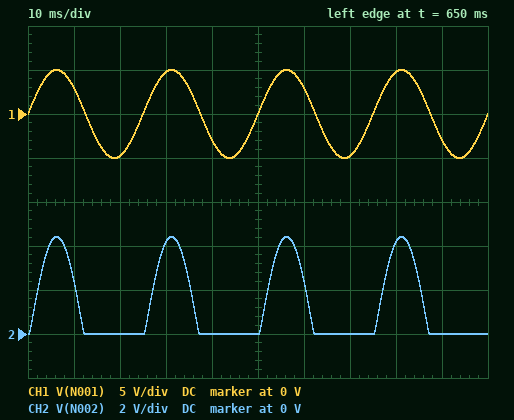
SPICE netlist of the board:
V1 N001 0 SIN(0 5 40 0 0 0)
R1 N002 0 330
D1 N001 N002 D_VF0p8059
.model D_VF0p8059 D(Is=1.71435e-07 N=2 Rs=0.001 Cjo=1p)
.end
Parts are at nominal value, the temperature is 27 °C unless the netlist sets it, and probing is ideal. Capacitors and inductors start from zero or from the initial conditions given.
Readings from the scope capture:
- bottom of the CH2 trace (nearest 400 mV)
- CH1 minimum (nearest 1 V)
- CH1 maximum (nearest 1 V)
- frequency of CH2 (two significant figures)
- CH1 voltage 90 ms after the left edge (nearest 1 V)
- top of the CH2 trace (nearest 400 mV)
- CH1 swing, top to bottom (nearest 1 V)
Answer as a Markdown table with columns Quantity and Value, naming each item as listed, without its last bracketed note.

| Quantity | Value |
|---|---|
| bottom of the CH2 trace | 0 V |
| CH1 minimum | -5 V |
| CH1 maximum | 5 V |
| frequency of CH2 | 40 Hz |
| CH1 voltage 90 ms after the left edge | -3 V |
| top of the CH2 trace | 4.4 V |
| CH1 swing, top to bottom | 10 V |
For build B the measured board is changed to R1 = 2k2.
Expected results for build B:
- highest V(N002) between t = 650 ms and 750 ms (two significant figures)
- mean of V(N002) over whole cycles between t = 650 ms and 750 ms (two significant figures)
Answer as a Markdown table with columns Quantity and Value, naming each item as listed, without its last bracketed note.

| Quantity | Value |
|---|---|
| highest V(N002) between t = 650 ms and 750 ms | 4.5 V |
| mean of V(N002) over whole cycles between t = 650 ms and 750 ms | 1.4 V |
